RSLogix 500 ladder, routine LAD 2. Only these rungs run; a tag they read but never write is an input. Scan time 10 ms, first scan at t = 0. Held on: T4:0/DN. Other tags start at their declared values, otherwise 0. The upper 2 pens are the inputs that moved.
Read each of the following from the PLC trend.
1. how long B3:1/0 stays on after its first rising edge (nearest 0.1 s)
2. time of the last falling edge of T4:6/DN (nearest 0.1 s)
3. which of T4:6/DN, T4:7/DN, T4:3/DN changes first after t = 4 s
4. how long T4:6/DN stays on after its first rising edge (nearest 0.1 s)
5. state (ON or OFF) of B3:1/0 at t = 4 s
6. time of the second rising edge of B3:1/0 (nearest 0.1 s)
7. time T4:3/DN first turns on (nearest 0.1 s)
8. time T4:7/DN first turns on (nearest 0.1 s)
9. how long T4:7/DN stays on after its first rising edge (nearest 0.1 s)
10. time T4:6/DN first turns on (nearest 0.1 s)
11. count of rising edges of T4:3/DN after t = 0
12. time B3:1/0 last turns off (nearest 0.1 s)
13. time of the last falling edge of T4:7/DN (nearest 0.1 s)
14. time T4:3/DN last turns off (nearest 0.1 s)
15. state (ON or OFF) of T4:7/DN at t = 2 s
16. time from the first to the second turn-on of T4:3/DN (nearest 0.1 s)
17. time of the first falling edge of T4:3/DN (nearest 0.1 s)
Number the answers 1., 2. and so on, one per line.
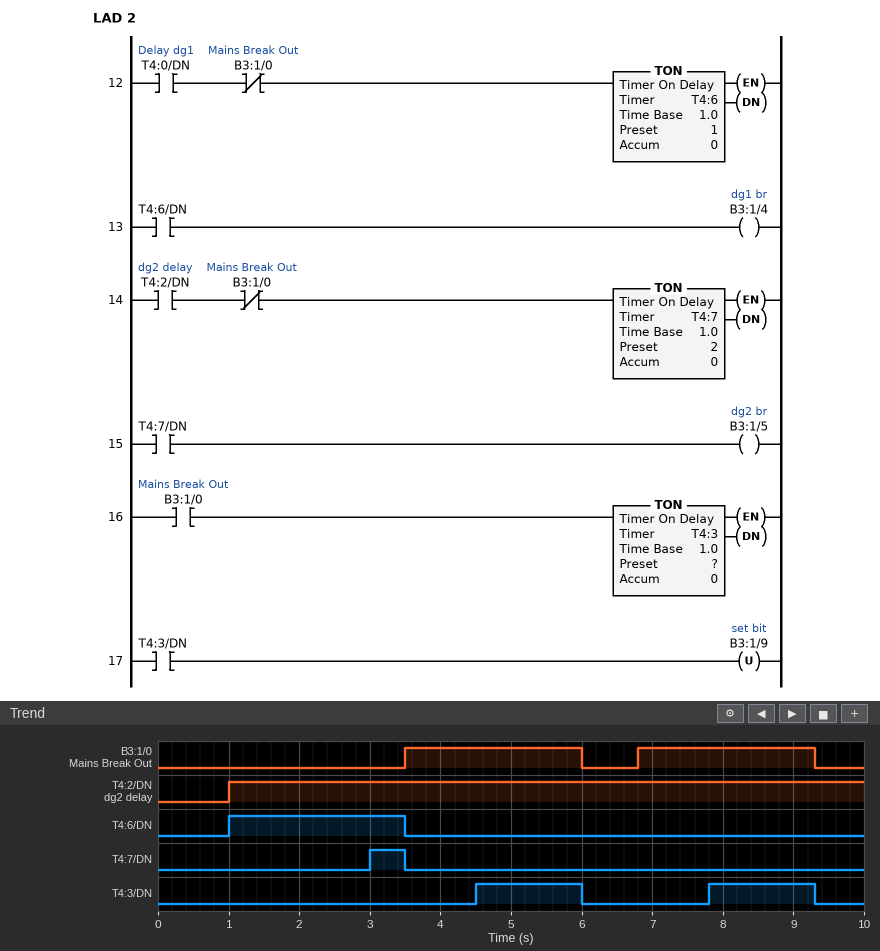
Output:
1. 2.5 s
2. 3.5 s
3. T4:3/DN
4. 2.5 s
5. ON
6. 6.8 s
7. 4.5 s
8. 3.0 s
9. 0.5 s
10. 1.0 s
11. 2
12. 9.3 s
13. 3.5 s
14. 9.3 s
15. OFF
16. 3.3 s
17. 6.0 s
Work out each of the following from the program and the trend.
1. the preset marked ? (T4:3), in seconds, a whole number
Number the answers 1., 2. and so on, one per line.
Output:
1. 1 s
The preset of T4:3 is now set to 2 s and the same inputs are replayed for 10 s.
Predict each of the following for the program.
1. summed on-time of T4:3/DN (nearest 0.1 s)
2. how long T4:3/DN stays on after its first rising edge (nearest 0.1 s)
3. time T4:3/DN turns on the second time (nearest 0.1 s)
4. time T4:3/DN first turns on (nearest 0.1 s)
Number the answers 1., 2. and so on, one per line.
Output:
1. 1.0 s
2. 0.5 s
3. 8.8 s
4. 5.5 s
